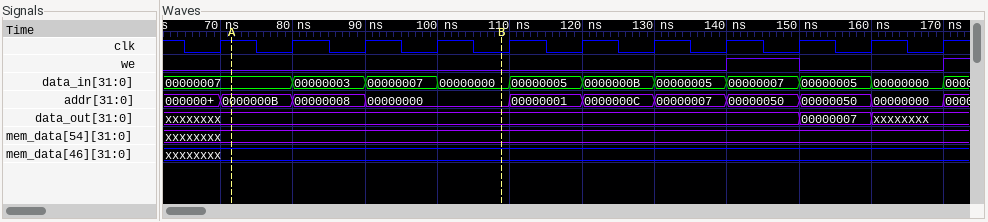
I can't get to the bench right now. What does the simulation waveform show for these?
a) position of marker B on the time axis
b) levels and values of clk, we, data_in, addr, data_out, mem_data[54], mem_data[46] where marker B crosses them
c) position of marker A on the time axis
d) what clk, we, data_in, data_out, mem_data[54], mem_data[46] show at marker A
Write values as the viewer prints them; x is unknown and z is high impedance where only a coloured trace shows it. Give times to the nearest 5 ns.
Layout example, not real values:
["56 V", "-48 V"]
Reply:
["110 ns", "clk=0, we=0, data_in=00000000, addr=00000000, data_out=xxxxxxxx, mem_data[54]=xxxxxxxx, mem_data[46]=xxxxxxxx", "70 ns", "clk=1, we=0, data_in=00000007, data_out=xxxxxxxx, mem_data[54]=xxxxxxxx, mem_data[46]=xxxxxxxx"]
